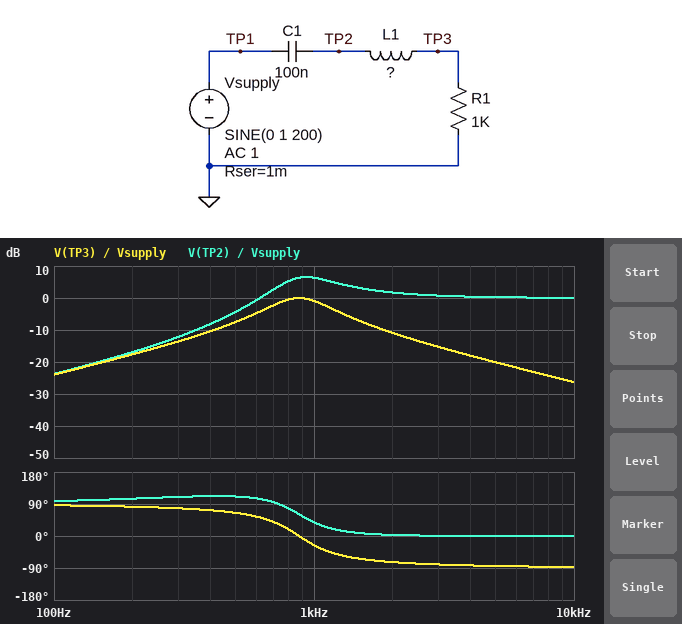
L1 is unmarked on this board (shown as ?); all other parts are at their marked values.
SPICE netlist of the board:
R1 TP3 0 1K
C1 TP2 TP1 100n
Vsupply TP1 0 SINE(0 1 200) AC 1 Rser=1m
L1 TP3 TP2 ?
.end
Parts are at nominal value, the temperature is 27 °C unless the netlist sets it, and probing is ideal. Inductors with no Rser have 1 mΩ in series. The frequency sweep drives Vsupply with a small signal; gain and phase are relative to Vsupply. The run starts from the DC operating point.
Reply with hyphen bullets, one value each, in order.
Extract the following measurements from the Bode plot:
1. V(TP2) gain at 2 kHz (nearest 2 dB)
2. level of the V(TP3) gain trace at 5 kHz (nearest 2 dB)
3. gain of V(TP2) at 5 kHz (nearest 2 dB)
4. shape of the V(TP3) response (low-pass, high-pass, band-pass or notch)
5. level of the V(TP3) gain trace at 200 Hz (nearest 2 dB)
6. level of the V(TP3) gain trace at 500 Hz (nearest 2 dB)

- 2 dB
- -20 dB
- 0 dB
- band-pass
- -18 dB
- -8 dB
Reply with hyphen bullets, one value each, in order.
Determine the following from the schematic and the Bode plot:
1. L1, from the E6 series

- 330 mH
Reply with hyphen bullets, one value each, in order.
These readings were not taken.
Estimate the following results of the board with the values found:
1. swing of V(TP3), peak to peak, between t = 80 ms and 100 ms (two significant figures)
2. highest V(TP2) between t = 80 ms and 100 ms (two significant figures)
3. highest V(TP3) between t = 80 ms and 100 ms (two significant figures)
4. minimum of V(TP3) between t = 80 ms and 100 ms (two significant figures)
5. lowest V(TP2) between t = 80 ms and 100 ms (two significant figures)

- 260 mV
- 140 mV
- 130 mV
- -130 mV
- -140 mV
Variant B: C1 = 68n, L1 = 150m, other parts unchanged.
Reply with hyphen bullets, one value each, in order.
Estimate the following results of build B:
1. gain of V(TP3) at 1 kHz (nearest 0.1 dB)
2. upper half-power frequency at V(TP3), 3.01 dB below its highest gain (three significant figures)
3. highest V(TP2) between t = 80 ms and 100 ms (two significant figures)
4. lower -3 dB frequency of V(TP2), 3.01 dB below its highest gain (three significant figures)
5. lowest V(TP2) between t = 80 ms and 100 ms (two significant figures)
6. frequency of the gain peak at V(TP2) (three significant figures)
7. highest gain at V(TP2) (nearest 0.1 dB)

- -4.7 dB
- 2.19 kHz
- 88 mV
- 1.27 kHz
- -88 mV
- 1.72 kHz
- 5.3 dB
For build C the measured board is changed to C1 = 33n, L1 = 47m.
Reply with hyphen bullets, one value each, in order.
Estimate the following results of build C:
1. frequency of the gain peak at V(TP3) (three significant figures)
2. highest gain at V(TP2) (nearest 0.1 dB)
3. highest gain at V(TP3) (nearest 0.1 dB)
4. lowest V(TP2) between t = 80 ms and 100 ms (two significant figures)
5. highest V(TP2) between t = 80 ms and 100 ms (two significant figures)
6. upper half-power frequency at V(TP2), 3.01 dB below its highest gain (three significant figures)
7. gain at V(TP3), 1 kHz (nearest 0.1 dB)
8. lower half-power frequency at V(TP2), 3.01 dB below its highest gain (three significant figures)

- 4.04 kHz
- 4.1 dB
- 0 dB
- -42 mV
- 42 mV
- 11.0 kHz
- -13.3 dB
- 3.10 kHz
